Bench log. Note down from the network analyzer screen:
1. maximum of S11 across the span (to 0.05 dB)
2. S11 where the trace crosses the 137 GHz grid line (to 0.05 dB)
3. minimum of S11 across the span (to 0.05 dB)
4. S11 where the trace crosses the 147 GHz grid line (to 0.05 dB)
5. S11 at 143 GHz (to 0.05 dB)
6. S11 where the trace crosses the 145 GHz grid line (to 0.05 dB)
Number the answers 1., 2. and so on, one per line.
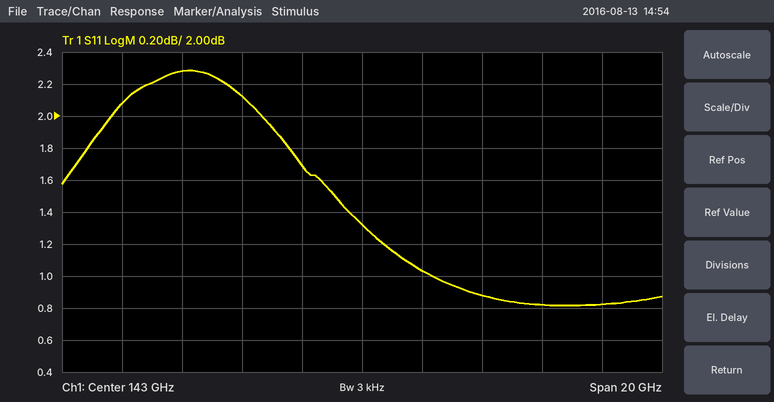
1. 2.30 dB
2. 2.30 dB
3. 0.80 dB
4. 0.90 dB
5. 1.30 dB
6. 1.05 dB
